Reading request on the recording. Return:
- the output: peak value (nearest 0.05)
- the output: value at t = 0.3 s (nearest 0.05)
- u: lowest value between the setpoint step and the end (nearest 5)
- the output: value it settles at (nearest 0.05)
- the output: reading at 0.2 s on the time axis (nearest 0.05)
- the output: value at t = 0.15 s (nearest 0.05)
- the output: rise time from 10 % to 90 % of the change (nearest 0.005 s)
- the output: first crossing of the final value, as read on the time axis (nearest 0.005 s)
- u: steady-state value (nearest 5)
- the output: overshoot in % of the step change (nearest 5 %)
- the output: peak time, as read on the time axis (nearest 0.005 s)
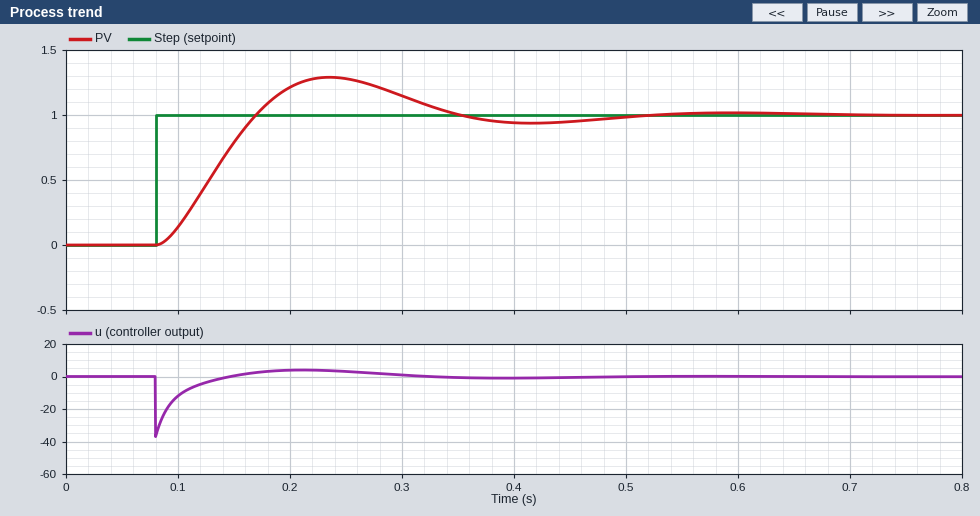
1.30
1.15
-35
1.00
1.20
0.80
0.065 s
0.170 s
0
30 %
0.235 s
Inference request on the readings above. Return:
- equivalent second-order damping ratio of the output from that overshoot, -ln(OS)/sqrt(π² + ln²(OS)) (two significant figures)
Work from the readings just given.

0.36
